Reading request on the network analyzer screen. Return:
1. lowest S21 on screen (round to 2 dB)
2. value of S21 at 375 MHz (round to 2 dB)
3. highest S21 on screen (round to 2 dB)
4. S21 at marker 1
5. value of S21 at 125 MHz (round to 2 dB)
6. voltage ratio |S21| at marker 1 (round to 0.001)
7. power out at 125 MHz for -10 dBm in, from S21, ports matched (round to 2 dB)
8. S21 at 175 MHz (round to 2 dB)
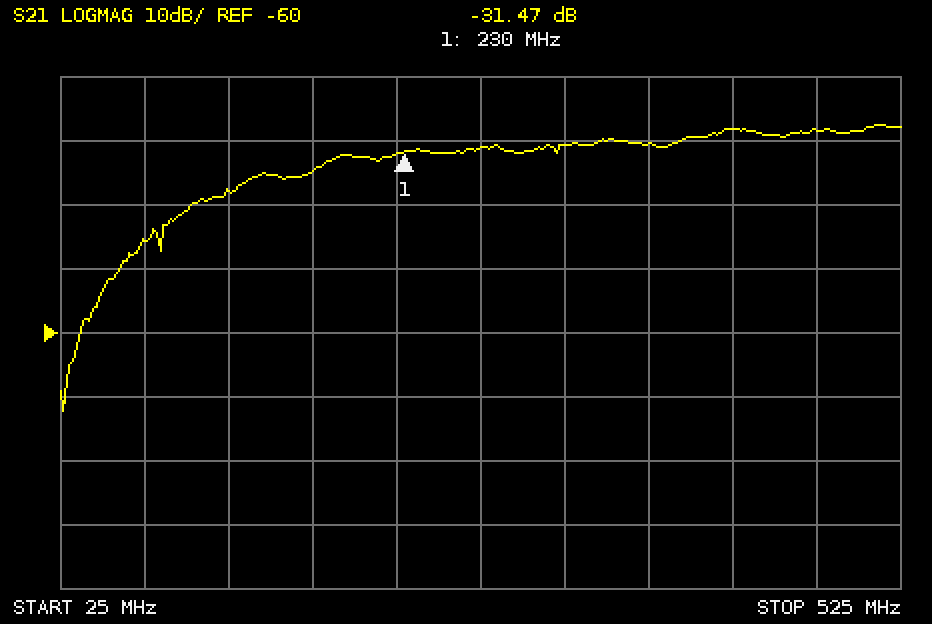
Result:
-72 dB
-30 dB
-28 dB
-31.47 dB
-38 dB
0.027
-48 dBm
-34 dB
